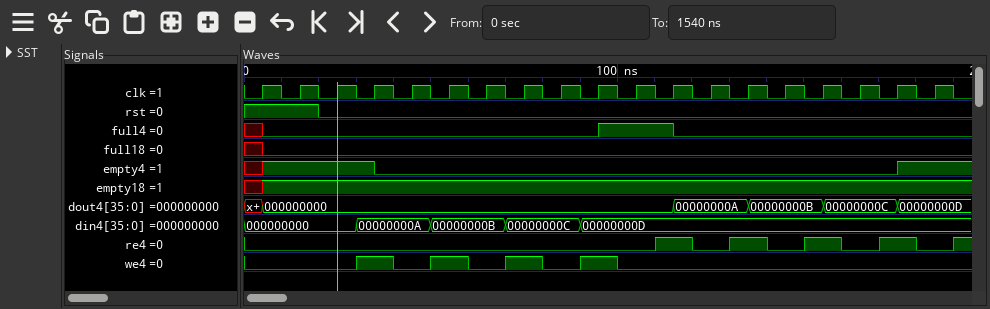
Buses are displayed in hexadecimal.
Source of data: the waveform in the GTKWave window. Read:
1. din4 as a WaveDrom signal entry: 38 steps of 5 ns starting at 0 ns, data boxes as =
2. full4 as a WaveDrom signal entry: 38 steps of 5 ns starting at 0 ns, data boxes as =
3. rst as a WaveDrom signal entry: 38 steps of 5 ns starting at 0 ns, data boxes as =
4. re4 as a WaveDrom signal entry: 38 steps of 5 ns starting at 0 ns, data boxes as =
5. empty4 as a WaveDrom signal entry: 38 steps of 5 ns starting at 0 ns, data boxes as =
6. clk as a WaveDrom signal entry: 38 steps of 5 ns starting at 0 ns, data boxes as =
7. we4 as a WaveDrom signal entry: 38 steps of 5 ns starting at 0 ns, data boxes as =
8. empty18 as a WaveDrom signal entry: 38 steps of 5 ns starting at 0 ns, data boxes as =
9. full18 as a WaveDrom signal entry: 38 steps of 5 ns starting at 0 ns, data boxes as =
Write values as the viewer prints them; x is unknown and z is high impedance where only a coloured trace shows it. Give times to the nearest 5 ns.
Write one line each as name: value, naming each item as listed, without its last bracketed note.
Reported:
din4 as a WaveDrom signal entry: 38 steps of 5 ns starting at 0 ns, data boxes as =: {name: 'din4', wave: '=.....=...=...=...=...................', data: '000000000 00000000A 00000000B 00000000C 00000000D'}
full4 as a WaveDrom signal entry: 38 steps of 5 ns starting at 0 ns, data boxes as =: {name: 'full4', wave: 'x0.................1...0..............'}
rst as a WaveDrom signal entry: 38 steps of 5 ns starting at 0 ns, data boxes as =: {name: 'rst', wave: '1...0.................................'}
re4 as a WaveDrom signal entry: 38 steps of 5 ns starting at 0 ns, data boxes as =: {name: 're4', wave: '0.....................1.0.1.0.1.0.1.0.'}
empty4 as a WaveDrom signal entry: 38 steps of 5 ns starting at 0 ns, data boxes as =: {name: 'empty4', wave: 'x1.....0...........................1..'}
clk as a WaveDrom signal entry: 38 steps of 5 ns starting at 0 ns, data boxes as =: {name: 'clk', wave: '01010101010101010101010101010101010101'}
we4 as a WaveDrom signal entry: 38 steps of 5 ns starting at 0 ns, data boxes as =: {name: 'we4', wave: '0.....1.0.1.0.1.0.1.0.................'}
empty18 as a WaveDrom signal entry: 38 steps of 5 ns starting at 0 ns, data boxes as =: {name: 'empty18', wave: 'x1....................................'}
full18 as a WaveDrom signal entry: 38 steps of 5 ns starting at 0 ns, data boxes as =: {name: 'full18', wave: 'x0....................................'}
